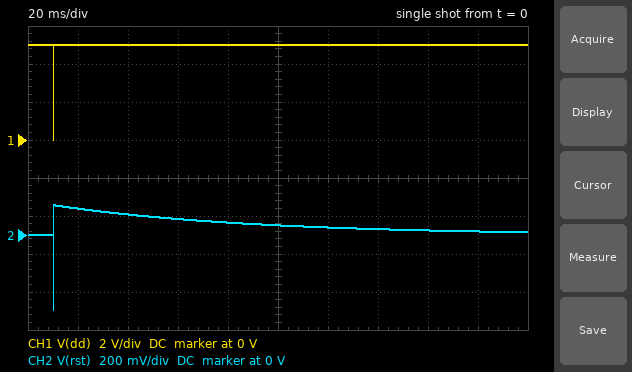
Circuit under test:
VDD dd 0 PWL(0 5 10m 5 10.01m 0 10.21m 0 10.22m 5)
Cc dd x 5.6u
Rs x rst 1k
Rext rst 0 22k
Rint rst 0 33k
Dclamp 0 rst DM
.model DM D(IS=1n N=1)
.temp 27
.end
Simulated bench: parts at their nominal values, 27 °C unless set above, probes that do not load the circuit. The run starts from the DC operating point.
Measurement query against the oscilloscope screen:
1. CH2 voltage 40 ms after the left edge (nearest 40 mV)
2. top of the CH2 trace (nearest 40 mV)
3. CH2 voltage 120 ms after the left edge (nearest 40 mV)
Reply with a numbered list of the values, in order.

1. 120 mV
2. 160 mV
3. 40 mV
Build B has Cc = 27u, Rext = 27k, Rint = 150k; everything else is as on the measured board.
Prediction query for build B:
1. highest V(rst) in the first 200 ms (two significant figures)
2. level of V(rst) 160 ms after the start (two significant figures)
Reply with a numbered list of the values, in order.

1. 34 mV
2. 27 mV
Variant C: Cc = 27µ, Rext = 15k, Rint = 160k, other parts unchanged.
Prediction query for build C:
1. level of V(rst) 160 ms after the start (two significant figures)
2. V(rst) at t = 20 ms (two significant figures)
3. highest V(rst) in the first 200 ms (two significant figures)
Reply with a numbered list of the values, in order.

1. 23 mV
2. 32 mV
3. 33 mV
